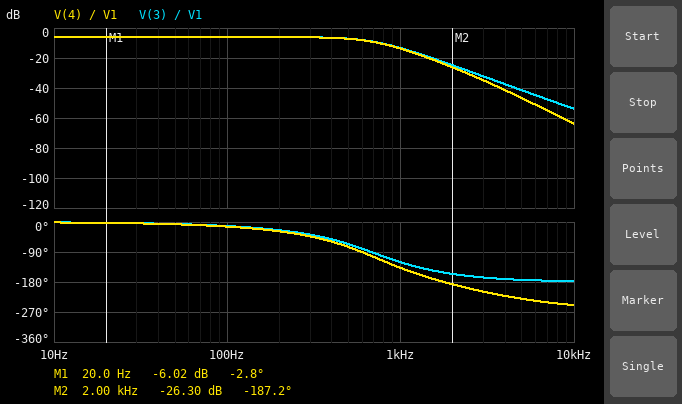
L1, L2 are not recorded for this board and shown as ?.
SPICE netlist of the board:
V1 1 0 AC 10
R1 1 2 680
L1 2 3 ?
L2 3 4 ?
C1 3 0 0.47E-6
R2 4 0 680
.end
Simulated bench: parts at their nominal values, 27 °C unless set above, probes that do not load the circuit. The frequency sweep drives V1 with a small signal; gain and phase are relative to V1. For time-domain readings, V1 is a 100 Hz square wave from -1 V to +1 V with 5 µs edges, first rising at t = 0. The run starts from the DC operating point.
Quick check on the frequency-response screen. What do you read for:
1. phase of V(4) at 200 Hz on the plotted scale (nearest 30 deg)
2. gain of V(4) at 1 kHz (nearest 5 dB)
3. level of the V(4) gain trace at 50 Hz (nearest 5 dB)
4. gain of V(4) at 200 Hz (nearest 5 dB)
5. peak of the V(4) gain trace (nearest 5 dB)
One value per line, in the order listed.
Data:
-30 deg
-15 dB
-5 dB
-5 dB
-5 dB
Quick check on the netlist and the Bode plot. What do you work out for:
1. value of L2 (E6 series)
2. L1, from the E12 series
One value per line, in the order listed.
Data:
33 mH
270 mH
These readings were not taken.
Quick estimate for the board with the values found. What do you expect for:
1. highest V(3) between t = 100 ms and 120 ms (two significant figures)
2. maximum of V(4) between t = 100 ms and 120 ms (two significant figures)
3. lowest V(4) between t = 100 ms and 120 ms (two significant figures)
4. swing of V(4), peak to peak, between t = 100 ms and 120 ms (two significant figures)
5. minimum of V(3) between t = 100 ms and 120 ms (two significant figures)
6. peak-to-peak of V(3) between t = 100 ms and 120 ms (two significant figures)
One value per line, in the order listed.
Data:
540 mV
540 mV
-540 mV
1.1 V
-540 mV
1.1 V
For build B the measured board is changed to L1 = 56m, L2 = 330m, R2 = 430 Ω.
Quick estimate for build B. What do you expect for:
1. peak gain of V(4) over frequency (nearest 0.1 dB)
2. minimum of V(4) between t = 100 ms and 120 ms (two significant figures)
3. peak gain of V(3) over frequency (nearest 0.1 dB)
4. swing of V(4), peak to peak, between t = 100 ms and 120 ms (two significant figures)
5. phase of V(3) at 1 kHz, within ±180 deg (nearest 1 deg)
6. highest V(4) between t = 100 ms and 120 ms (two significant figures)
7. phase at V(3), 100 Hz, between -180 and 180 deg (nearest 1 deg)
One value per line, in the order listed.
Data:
-8.2 dB
-420 mV
-1.7 dB
840 mV
-84 deg
420 mV
9 deg
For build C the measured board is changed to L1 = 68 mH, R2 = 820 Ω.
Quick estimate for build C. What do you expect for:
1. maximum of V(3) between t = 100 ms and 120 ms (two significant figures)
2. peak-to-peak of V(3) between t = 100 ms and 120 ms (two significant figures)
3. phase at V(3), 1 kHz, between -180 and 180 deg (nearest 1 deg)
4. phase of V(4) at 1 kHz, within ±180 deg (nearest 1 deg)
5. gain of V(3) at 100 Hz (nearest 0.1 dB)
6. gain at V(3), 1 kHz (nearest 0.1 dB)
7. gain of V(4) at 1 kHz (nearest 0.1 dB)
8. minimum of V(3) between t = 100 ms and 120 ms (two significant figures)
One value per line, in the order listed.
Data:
570 mV
1.1 V
-74 deg
-89 deg
-5.3 dB
-7.6 dB
-7.8 dB
-570 mV
